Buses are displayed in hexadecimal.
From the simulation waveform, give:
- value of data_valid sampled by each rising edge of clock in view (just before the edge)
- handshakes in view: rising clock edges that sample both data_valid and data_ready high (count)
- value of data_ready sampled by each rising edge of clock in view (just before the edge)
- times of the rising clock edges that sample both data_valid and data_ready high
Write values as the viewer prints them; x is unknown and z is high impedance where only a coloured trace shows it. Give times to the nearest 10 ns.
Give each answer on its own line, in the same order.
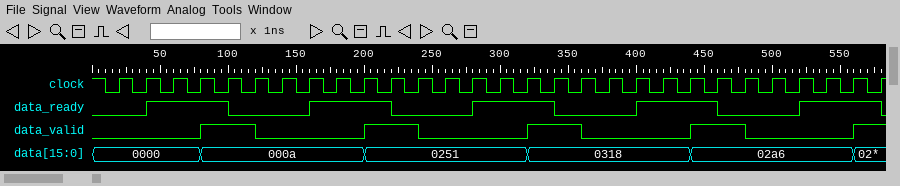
0 0 0 0 1 1 0 0 0 0 1 1 0 0 0 0 1 1 0 0 0 0 1 1 0 0 0 0 1
5
0 0 1 1 1 0 0 0 1 1 1 0 0 0 1 1 1 0 0 0 1 1 1 0 0 0 1 1 1
100 ns, 220 ns, 340 ns, 460 ns, 580 ns
